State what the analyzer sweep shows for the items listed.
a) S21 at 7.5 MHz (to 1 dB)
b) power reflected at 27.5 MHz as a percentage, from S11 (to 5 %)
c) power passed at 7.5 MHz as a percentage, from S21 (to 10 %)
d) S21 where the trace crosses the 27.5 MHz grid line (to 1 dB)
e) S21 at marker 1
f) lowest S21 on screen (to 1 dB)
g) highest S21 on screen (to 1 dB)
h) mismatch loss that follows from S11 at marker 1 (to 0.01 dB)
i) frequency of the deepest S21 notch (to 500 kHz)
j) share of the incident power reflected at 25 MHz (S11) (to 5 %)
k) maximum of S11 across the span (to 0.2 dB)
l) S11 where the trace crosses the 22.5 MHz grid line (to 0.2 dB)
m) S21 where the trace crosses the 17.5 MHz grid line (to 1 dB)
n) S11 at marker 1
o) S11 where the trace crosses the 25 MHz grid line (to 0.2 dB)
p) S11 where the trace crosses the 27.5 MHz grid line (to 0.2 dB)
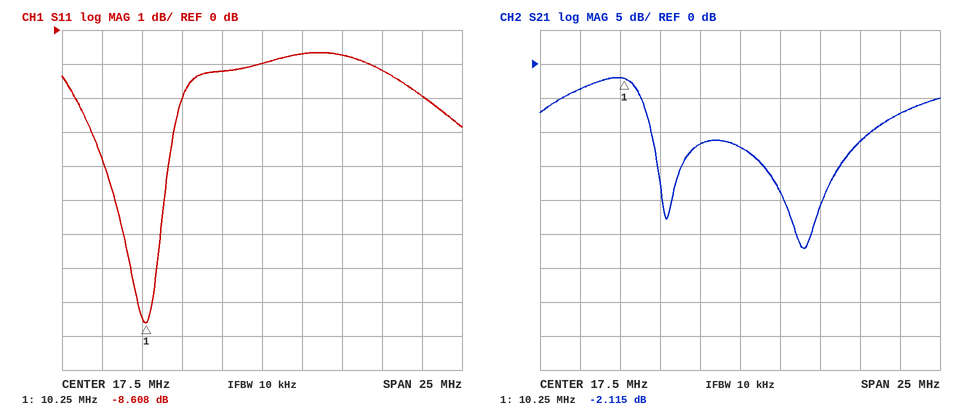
-4 dB
65 %
40 %
-7 dB
-2.115 dB
-27 dB
-2 dB
0.64 dB
21.5 MHz
75 %
-0.6 dB
-0.8 dB
-12 dB
-8.608 dB
-1.2 dB
-2.0 dB
